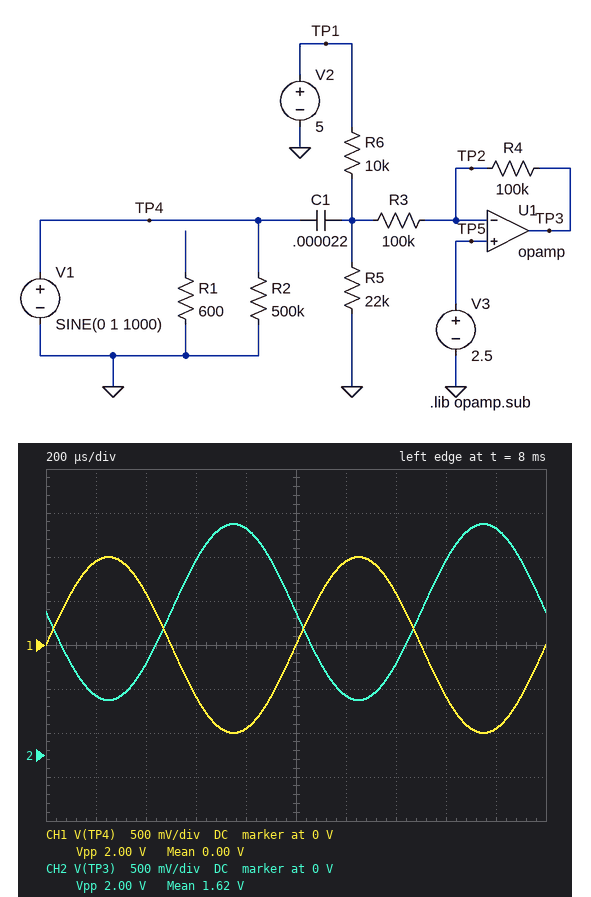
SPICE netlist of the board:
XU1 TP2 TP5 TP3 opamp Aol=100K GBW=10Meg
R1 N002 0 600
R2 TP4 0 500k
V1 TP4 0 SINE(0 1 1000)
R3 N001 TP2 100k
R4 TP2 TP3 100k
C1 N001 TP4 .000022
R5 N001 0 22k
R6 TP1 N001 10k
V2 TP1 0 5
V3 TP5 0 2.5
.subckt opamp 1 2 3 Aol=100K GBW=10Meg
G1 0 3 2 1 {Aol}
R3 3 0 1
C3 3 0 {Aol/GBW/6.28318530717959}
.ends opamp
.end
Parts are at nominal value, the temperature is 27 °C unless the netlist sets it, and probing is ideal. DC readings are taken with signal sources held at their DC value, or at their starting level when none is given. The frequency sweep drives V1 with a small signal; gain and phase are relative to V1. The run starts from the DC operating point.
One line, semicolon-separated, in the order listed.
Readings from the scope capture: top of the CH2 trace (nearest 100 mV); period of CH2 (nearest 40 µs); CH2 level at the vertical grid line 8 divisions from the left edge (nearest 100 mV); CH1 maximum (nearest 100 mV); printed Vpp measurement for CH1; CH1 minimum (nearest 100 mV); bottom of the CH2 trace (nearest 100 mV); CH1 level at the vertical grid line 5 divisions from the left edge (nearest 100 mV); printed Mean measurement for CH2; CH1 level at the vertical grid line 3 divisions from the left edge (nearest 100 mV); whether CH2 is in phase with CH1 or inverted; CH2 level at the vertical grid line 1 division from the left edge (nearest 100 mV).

2.6 V; 1.00 ms; 2.2 V; 1.0 V; 2.00 V; -1.0 V; 600 mV; 0 V; 1.62 V; -600 mV; inverted; 700 mV
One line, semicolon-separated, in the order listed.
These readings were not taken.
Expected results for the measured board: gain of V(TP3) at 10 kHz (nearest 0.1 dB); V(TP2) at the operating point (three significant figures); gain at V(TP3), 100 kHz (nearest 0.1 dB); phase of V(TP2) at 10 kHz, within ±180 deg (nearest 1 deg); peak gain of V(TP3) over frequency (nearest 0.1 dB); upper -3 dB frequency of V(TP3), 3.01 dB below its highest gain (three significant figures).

0 dB; 2.50 V; 0 dB; 89 deg; 0 dB; 5.00 MHz
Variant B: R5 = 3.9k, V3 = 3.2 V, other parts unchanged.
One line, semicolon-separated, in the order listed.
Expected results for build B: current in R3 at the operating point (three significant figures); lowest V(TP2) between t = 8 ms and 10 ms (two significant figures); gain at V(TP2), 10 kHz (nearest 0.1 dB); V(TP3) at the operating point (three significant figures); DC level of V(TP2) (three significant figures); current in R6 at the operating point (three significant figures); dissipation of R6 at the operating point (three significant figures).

17.5 µA; 3.2 V; -60.0 dB; 4.95 V; 3.20 V; 355 µA; 1.26 mW
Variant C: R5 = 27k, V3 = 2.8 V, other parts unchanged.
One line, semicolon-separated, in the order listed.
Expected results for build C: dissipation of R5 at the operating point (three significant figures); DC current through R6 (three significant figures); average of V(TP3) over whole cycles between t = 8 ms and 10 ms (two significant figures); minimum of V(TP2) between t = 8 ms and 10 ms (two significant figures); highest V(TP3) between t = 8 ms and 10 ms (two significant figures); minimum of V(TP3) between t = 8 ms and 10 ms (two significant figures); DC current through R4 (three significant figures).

478 µW; 141 µA; 2.0 V; 2.8 V; 3.0 V; 1.0 V; 7.91 µA
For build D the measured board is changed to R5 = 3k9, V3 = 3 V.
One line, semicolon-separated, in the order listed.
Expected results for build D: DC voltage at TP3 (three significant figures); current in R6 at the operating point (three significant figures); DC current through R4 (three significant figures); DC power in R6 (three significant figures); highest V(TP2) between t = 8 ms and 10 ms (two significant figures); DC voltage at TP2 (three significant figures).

4.55 V; 355 µA; 15.5 µA; 1.26 mW; 3.0 V; 3.00 V
